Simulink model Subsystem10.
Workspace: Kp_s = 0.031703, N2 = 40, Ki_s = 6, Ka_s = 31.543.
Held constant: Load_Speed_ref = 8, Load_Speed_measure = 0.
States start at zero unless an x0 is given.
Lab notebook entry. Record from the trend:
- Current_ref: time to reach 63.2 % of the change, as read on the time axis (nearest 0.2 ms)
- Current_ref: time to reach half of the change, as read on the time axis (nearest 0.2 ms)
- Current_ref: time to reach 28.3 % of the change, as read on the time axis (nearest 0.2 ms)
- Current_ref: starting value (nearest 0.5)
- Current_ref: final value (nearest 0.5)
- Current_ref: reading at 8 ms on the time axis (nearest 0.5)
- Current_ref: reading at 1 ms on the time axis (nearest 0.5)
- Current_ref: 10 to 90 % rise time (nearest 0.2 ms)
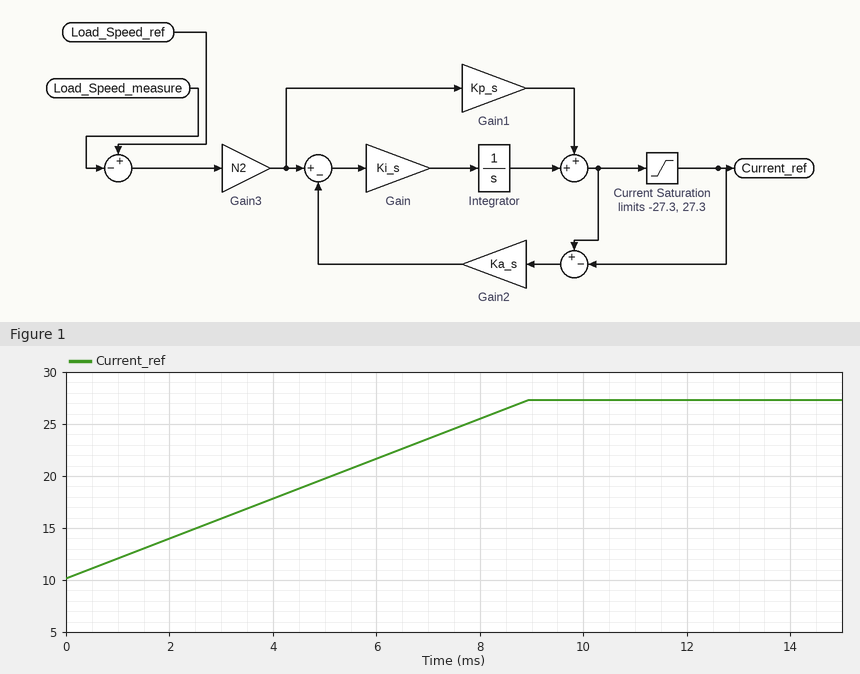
5.6 ms
4.4 ms
2.6 ms
10.0
27.5
25.5
12.0
7.2 ms
